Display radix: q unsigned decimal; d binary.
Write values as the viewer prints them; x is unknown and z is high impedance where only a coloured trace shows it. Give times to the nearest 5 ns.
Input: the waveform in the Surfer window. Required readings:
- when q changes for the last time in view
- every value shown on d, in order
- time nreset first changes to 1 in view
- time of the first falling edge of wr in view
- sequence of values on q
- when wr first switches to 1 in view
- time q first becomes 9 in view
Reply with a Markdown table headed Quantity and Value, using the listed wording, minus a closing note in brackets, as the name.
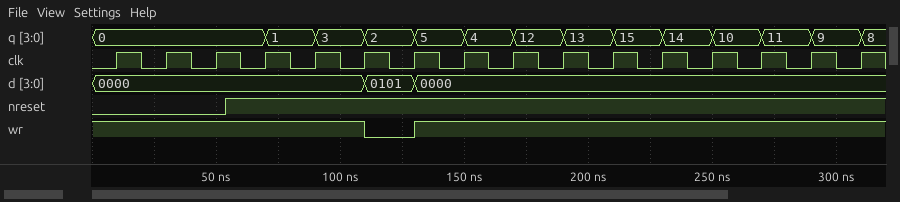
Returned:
| Quantity | Value |
|---|---|
| when q changes for the last time in view | 310 ns |
| every value shown on d, in order | 0000, 0101, 0000 |
| time nreset first changes to 1 in view | 55 ns |
| time of the first falling edge of wr in view | 110 ns |
| sequence of values on q | 0, 1, 3, 2, 5, 4, 12, 13, 15, 14, 10, 11, 9, 8 |
| when wr first switches to 1 in view | 130 ns |
| time q first becomes 9 in view | 290 ns |
